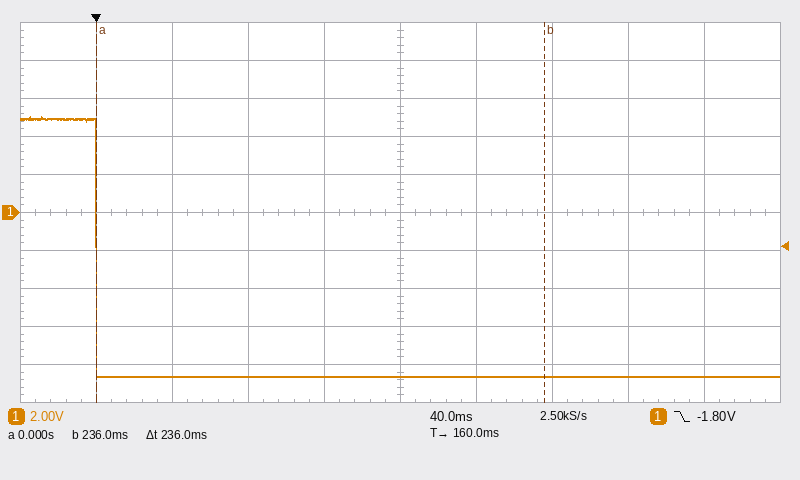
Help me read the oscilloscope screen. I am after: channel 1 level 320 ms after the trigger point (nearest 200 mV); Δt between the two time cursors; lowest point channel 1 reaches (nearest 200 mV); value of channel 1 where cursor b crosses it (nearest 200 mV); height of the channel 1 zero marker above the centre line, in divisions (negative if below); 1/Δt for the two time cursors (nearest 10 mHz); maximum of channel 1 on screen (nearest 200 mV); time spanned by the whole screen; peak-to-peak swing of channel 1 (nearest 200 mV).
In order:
-8.6 V
236 ms
-8.6 V
-8.6 V
0.0 div
4.24 Hz
5.0 V
400 ms
13.6 V
